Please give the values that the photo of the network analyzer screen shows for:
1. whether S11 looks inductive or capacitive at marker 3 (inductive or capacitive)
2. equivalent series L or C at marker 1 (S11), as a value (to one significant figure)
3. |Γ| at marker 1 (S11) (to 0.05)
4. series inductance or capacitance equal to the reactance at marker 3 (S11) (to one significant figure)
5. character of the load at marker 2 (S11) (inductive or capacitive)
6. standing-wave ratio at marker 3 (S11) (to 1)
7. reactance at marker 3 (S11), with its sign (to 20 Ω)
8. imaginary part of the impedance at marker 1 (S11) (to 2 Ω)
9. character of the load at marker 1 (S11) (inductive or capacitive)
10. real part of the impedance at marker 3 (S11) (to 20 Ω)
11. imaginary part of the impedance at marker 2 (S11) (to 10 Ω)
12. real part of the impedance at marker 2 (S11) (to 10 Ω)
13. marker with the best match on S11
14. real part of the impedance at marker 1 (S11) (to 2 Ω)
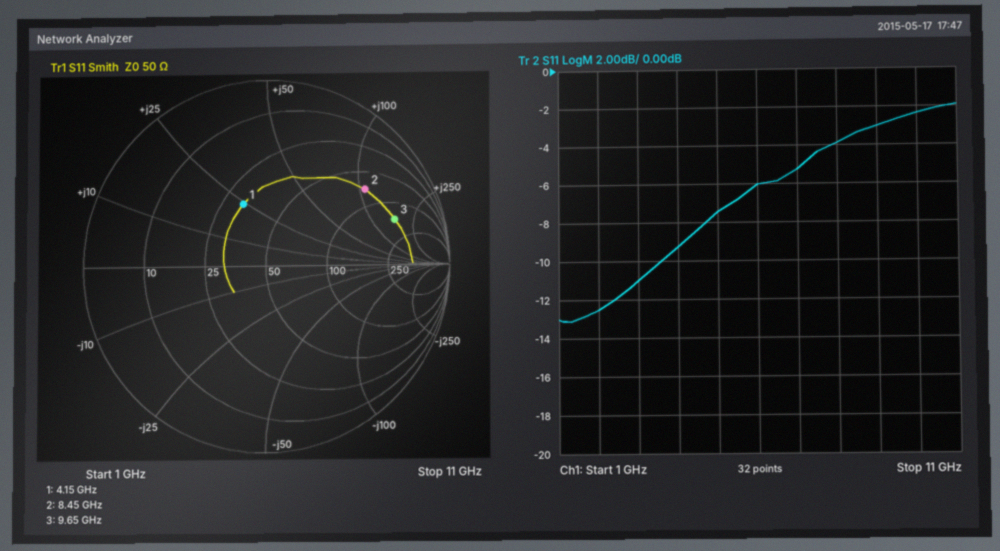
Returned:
inductive
900 pH
0.35
3 nH
inductive
7
+160 Ω
+24 Ω
inductive
160 Ω
+110 Ω
70 Ω
marker 1
32 Ω
